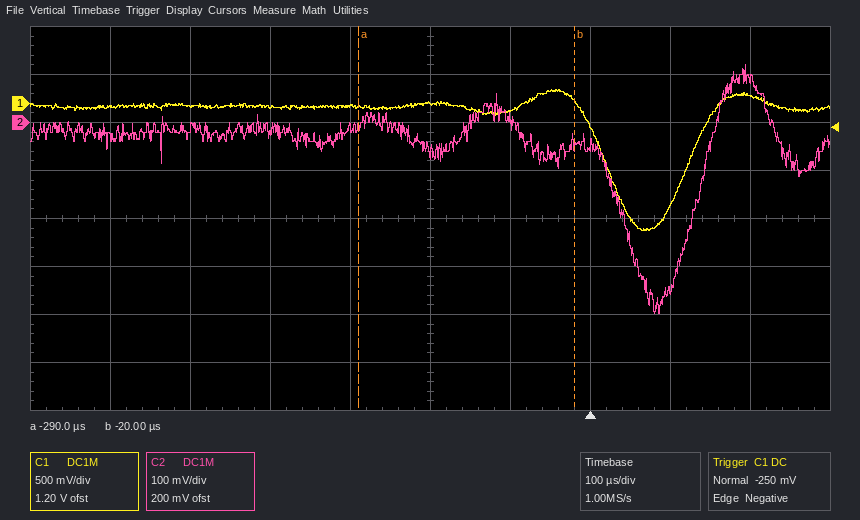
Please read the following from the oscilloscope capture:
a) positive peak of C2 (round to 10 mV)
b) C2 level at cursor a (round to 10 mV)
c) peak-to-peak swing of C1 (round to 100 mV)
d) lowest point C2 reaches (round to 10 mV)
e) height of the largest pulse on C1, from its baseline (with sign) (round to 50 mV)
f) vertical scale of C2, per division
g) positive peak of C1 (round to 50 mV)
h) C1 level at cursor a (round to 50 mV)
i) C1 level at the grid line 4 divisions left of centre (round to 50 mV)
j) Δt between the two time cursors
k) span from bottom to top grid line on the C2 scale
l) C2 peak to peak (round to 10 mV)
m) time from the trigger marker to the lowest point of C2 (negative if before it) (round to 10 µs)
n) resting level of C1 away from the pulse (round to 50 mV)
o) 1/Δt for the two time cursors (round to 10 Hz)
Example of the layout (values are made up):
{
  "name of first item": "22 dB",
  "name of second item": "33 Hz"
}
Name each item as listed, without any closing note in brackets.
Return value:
{
  "positive peak of C2": "120 mV",
  "C2 level at cursor a": "-10 mV",
  "peak-to-peak swing of C1": "1.50 V",
  "lowest point C2 reaches": "-400 mV",
  "height of the largest pulse on C1, from its baseline (with sign)": "-1.30 V",
  "vertical scale of C2, per division": "100 mV",
  "positive peak of C1": "150 mV",
  "C1 level at cursor a": "-50 mV",
  "C1 level at the grid line 4 divisions left of centre": "-50 mV",
  "Δt between the two time cursors": "270 µs",
  "span from bottom to top grid line on the C2 scale": "800 mV",
  "C2 peak to peak": "520 mV",
  "time from the trigger marker to the lowest point of C2 (negative if before it)": "+80 µs",
  "resting level of C1 away from the pulse": "-50 mV",
  "1/Δt for the two time cursors": "3.70 kHz"
}
